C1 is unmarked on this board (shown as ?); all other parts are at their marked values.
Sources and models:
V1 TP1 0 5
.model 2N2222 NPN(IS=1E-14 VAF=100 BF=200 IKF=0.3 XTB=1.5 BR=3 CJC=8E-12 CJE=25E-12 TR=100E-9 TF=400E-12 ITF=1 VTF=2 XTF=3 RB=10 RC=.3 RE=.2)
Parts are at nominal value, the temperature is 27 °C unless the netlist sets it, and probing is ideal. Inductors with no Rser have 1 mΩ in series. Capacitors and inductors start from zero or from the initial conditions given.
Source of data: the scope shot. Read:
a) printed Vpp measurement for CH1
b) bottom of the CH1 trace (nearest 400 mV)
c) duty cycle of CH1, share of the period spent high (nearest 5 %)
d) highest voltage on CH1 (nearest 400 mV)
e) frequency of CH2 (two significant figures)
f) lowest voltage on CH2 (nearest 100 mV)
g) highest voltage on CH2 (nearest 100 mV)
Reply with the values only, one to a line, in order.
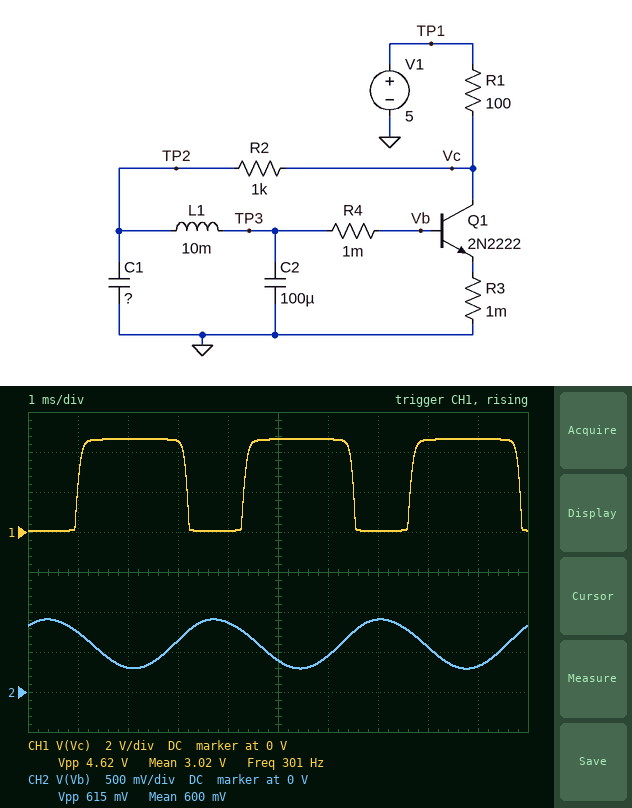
4.62 V
0 V
65 %
4.8 V
300 Hz
300 mV
900 mV
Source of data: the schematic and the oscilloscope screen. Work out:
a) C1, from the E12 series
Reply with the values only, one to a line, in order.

39 µF
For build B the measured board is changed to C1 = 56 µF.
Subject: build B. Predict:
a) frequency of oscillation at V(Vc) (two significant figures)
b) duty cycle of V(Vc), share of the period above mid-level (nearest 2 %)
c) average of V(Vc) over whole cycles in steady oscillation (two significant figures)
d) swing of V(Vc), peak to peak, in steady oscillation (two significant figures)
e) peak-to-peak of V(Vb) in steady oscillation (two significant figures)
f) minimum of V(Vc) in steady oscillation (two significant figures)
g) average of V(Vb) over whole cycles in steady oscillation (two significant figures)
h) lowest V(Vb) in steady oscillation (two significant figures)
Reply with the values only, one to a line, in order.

270 Hz
62 %
2.9 V
4.6 V
470 mV
60 mV
660 mV
420 mV
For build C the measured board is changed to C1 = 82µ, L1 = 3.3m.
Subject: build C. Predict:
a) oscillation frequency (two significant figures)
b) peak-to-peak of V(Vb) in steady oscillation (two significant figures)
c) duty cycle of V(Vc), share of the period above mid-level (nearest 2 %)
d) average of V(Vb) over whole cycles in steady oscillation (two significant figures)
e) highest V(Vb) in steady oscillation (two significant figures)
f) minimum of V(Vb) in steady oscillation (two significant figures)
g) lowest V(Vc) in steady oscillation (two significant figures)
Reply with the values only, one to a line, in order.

410 Hz
280 mV
56 %
720 mV
860 mV
580 mV
65 mV
